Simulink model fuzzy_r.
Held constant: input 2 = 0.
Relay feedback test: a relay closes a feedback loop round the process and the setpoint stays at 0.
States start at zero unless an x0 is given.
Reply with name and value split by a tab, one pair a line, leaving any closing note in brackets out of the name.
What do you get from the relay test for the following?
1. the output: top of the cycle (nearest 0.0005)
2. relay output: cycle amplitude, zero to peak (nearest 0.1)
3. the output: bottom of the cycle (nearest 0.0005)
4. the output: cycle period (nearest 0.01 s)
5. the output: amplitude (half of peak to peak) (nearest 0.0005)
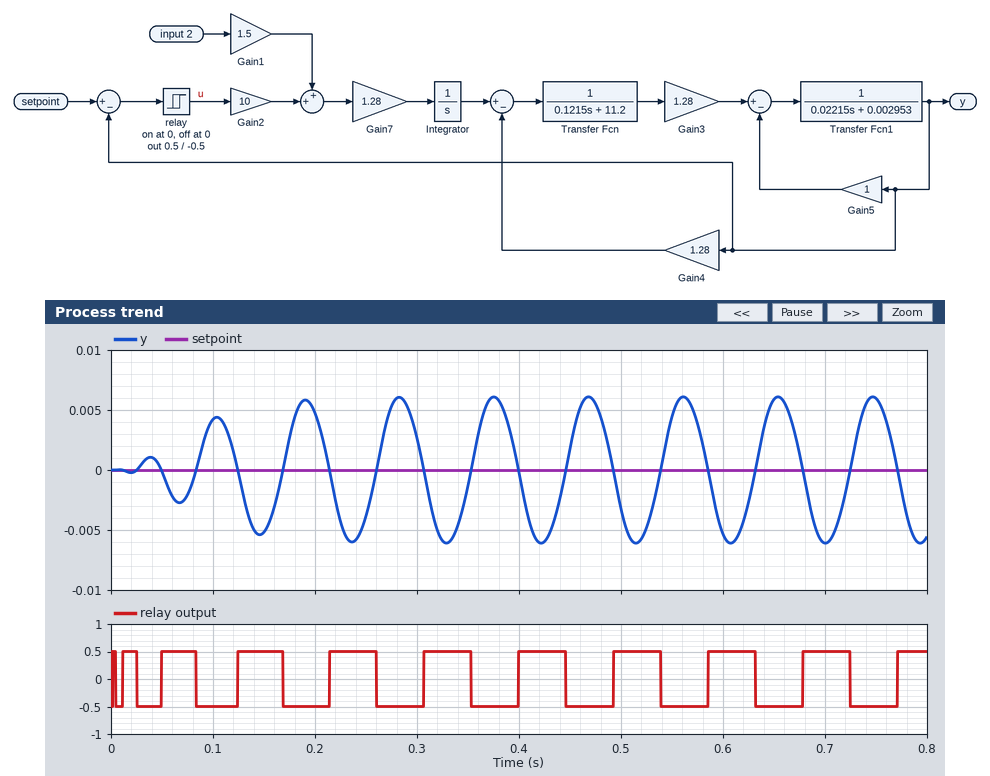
the output: top of the cycle	0.0060
relay output: cycle amplitude, zero to peak	0.5
the output: bottom of the cycle	-0.0060
the output: cycle period	0.09 s
the output: amplitude (half of peak to peak)	0.0060
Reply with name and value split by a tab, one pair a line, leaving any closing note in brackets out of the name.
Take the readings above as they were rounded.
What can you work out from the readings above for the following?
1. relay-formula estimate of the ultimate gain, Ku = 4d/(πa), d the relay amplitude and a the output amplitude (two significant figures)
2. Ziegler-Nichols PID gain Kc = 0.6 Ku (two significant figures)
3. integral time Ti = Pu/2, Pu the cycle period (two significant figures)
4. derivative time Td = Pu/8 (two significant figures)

relay-formula estimate of the ultimate gain, Ku = 4d/(πa), d the relay amplitude and a the output amplitude	110
Ziegler-Nichols PID gain Kc = 0.6 Ku	66
integral time Ti = Pu/2, Pu the cycle period	0.045 s
derivative time Td = Pu/8	0.011 s
